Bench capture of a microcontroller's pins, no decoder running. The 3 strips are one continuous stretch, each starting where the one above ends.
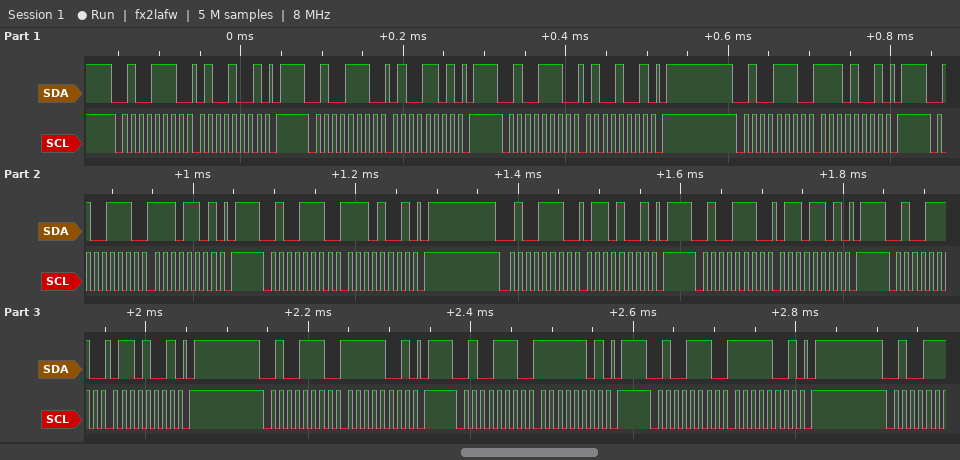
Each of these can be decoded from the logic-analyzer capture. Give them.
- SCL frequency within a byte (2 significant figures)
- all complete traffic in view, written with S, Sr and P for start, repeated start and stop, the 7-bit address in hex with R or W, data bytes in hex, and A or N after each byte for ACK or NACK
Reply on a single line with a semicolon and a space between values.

100 kHz; S 27W A 49 A P S 27W A 4D A P S 27W A 49 A P S 27W A E9 A P S 27W A ED A P S 27W A E9 A P S 27W A 69 A P S 27W A 6D A P S 27W A 69 A P S 27W A F9 A P S 27W A FD A P S 27W A F9 A P
